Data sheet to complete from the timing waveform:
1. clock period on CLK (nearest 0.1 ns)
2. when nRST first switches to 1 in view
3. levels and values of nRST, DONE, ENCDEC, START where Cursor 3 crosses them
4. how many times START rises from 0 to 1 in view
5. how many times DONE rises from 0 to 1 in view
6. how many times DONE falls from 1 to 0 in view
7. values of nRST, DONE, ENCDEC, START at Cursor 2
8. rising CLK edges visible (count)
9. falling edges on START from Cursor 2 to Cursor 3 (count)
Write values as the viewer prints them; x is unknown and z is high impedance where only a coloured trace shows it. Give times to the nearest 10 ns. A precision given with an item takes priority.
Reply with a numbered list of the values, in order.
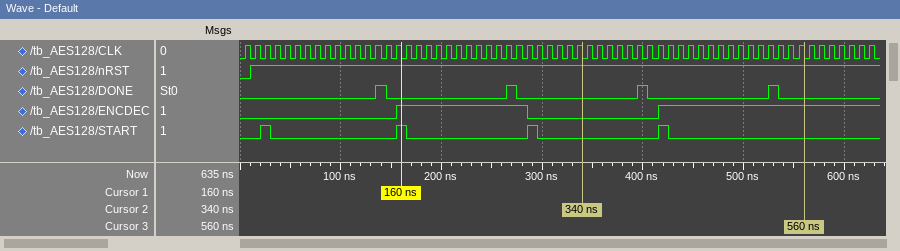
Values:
1. 10 ns
2. 10 ns
3. nRST=1, DONE=0, ENCDEC=1, START=0
4. 4
5. 4
6. 4
7. nRST=1, DONE=0, ENCDEC=0, START=0
8. 63
9. 1
